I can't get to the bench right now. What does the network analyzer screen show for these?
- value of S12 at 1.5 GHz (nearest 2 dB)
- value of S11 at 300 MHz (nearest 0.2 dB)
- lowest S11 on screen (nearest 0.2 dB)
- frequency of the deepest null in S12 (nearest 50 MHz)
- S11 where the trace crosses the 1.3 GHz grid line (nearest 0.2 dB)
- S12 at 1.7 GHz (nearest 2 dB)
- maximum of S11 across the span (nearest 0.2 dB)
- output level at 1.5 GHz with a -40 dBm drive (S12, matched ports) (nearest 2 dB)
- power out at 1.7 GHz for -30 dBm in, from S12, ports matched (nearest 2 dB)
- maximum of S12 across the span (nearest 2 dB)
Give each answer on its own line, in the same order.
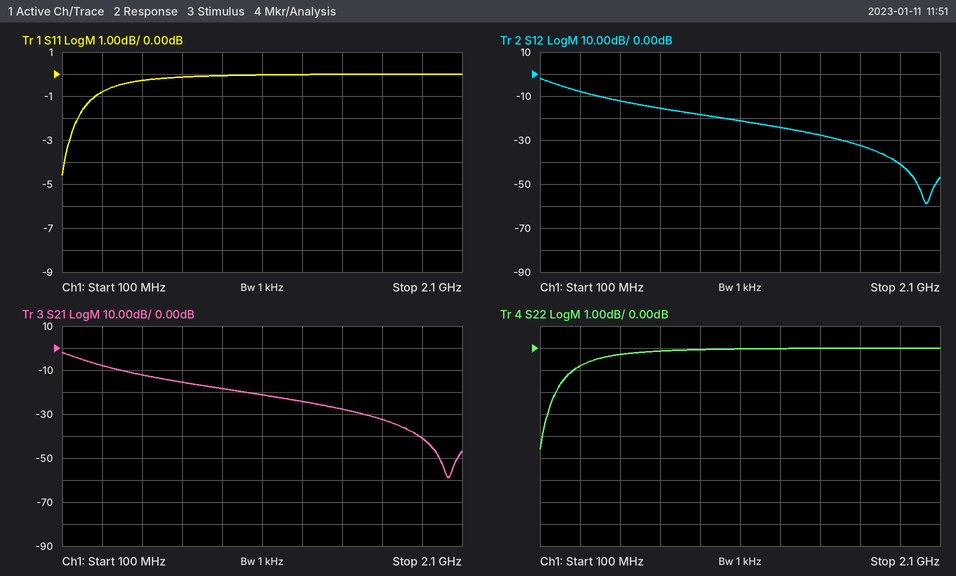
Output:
-28 dB
-0.8 dB
-4.6 dB
2.05 GHz
0.0 dB
-32 dB
0.0 dB
-68 dBm
-62 dBm
-2 dB
